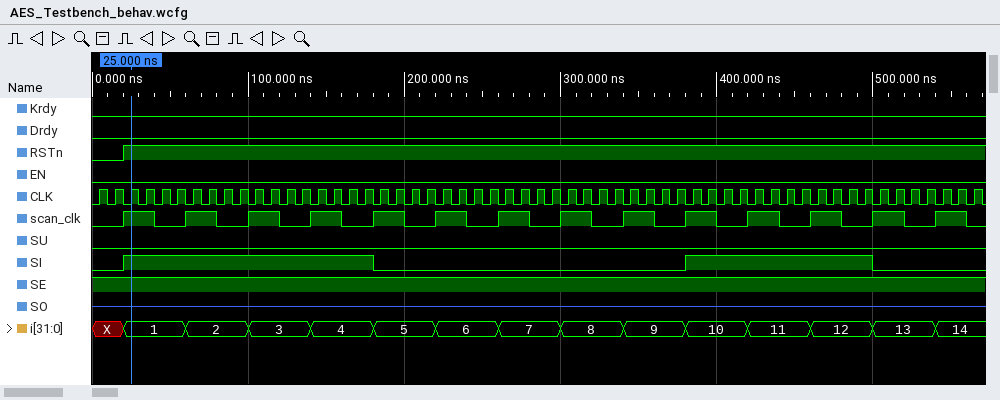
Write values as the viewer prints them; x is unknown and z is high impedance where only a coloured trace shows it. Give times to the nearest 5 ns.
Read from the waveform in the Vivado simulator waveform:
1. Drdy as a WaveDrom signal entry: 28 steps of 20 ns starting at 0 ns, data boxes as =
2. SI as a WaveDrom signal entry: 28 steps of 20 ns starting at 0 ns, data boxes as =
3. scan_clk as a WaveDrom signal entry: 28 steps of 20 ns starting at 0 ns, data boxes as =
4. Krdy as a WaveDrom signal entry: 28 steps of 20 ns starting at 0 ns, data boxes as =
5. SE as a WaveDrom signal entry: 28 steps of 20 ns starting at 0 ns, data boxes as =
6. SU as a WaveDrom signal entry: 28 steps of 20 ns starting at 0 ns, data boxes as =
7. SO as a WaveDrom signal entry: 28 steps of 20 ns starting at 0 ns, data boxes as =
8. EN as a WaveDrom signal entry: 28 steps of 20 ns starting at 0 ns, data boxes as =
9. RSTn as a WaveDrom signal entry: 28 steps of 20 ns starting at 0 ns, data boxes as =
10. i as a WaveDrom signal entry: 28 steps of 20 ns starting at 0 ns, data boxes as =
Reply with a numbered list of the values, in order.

1. {name: 'Drdy', wave: '0...........................'}
2. {name: 'SI', wave: '01.......0.........1.....0..'}
3. {name: 'scan_clk', wave: '0101010101010101010101010101'}
4. {name: 'Krdy', wave: '0...........................'}
5. {name: 'SE', wave: '1...........................'}
6. {name: 'SU', wave: '0...........................'}
7. {name: 'SO', wave: 'z...........................'}
8. {name: 'EN', wave: '0...........................'}
9. {name: 'RSTn', wave: '01..........................'}
10. {name: 'i', wave: 'x=.=.=.=.=.=.=.=.=.=.=.=.=.=', data: '1 2 3 4 5 6 7 8 9 10 11 12 13 14'}
